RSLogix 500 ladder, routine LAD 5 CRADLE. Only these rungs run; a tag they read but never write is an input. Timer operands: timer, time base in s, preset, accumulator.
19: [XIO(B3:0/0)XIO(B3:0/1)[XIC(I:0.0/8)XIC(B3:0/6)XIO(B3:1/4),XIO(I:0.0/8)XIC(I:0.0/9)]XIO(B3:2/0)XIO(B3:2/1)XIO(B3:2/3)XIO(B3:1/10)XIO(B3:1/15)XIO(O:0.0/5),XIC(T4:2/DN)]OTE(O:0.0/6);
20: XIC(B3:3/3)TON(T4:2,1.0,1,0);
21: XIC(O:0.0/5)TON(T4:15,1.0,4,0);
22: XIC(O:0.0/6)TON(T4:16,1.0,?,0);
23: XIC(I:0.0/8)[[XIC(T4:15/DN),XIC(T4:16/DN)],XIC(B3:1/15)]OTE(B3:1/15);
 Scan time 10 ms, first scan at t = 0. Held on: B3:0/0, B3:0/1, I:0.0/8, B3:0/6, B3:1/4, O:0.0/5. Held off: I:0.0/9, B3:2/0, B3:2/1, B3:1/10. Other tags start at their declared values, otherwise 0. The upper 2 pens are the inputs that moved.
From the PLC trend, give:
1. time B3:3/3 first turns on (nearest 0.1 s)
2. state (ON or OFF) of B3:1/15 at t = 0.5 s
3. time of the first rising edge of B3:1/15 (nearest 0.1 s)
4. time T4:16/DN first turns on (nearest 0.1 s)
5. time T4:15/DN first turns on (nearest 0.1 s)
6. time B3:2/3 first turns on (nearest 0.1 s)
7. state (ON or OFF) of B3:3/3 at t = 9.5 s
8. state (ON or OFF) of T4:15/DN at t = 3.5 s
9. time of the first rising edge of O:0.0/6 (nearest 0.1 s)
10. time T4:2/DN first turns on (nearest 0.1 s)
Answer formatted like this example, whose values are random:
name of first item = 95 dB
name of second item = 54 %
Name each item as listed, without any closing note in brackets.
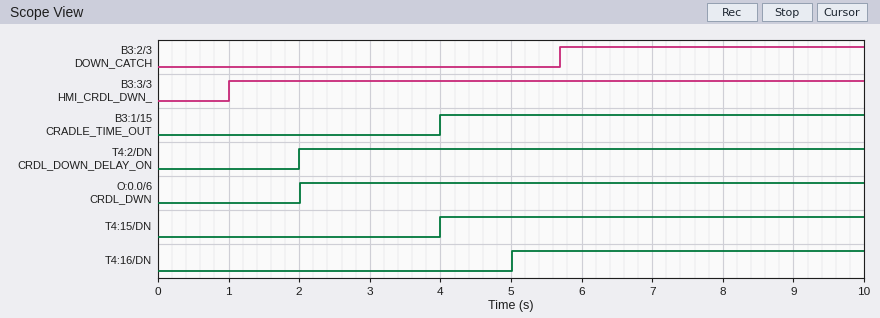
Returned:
time B3:3/3 first turns on = 1.0 s
state (ON or OFF) of B3:1/15 at t = 0.5 s = OFF
time of the first rising edge of B3:1/15 = 4.0 s
time T4:16/DN first turns on = 5.0 s
time T4:15/DN first turns on = 4.0 s
time B3:2/3 first turns on = 5.7 s
state (ON or OFF) of B3:3/3 at t = 9.5 s = ON
state (ON or OFF) of T4:15/DN at t = 3.5 s = OFF
time of the first rising edge of O:0.0/6 = 2.0 s
time T4:2/DN first turns on = 2.0 s
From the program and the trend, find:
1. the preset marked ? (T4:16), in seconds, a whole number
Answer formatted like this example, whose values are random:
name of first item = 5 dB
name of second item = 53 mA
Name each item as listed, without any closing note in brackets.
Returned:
the preset marked ? (T4:16), in seconds, a whole number = 3 s
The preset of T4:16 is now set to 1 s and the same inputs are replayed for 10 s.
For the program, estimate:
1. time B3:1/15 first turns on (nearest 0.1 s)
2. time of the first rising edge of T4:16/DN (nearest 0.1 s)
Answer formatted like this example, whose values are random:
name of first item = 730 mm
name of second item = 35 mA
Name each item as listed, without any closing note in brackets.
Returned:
time B3:1/15 first turns on = 3.0 s
time of the first rising edge of T4:16/DN = 3.0 s
